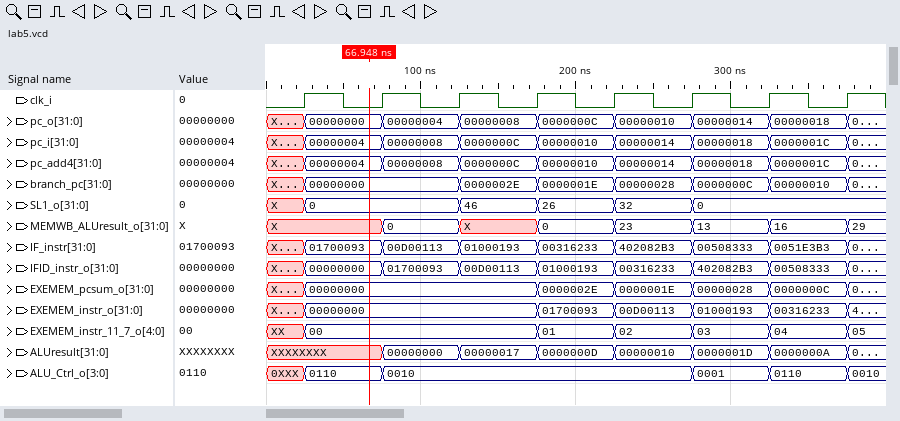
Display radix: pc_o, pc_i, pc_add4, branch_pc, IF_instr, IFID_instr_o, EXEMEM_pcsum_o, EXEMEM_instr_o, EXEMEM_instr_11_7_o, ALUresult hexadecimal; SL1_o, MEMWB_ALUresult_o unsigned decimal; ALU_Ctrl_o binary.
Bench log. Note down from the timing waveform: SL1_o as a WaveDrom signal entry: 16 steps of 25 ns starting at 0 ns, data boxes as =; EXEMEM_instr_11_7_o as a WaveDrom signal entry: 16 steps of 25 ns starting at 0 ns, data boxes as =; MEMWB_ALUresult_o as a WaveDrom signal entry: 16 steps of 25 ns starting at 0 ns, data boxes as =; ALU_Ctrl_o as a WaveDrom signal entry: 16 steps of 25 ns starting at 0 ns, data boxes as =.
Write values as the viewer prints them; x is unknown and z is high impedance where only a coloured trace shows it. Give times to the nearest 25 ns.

{name: 'SL1_o', wave: '==...=.=.=.=....', data: 'X 0 46 26 32 0'}
{name: 'EXEMEM_instr_11_7_o', wave: 'x=.....=.=.=.=.=', data: '00 01 02 03 04 05'}
{name: 'MEMWB_ALUresult_o', wave: 'x..=.x.=.=.=.=.=', data: '0 0 23 13 16 29'}
{name: 'ALU_Ctrl_o', wave: '==.=.......=.=.=', data: '0XXX 0110 0010 0001 0110 0010'}
